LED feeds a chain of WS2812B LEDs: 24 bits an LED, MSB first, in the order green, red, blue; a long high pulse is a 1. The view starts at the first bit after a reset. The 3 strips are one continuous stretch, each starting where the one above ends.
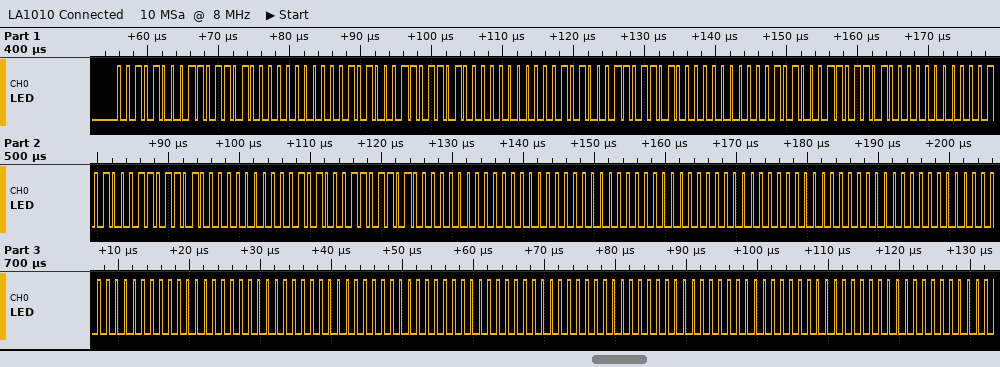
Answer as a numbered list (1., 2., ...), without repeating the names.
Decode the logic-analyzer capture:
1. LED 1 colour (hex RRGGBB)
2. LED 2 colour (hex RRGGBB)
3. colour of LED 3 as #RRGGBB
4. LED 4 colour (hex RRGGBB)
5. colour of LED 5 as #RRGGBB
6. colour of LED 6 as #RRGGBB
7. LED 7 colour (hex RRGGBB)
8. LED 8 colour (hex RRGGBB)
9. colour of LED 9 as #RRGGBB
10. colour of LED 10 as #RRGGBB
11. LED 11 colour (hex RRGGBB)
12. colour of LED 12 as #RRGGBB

1. #DA2800
2. #DA2800
3. #DA2800
4. #DA2800
5. #DA2800
6. #DA2800
7. #000000
8. #000000
9. #000000
10. #000000
11. #000000
12. #000000
